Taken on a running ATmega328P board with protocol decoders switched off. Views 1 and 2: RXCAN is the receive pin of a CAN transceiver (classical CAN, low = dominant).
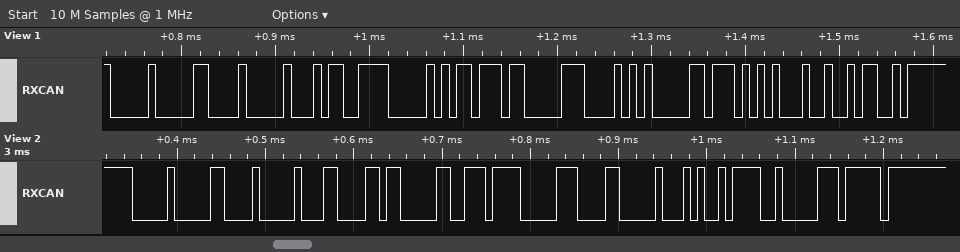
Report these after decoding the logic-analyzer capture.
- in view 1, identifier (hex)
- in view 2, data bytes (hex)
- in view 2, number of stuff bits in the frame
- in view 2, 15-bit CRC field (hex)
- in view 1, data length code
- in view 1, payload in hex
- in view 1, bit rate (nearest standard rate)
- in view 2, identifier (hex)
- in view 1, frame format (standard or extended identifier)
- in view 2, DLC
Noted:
0x002
06 1B 04 EF 06 18 05 2F
7
0x106F
8
05 9E 05 BB 06 15 05 D5
125 kbit/s
0x002
standard
8
